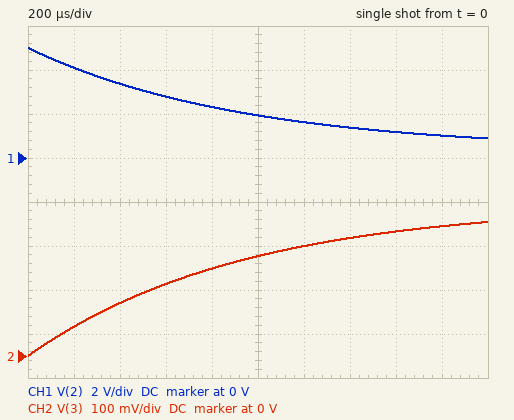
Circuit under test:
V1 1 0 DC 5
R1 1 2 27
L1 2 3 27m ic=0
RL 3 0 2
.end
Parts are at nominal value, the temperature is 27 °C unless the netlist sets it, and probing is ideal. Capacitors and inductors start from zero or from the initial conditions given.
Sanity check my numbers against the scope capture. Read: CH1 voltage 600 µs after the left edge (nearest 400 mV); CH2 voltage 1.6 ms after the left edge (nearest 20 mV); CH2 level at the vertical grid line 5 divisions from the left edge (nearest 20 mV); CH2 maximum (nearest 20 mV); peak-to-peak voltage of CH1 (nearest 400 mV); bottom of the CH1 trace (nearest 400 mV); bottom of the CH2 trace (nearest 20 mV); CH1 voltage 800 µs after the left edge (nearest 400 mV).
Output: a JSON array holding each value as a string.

["2.8 V", "280 mV", "220 mV", "300 mV", "4.0 V", "800 mV", "0 V", "2.4 V"]
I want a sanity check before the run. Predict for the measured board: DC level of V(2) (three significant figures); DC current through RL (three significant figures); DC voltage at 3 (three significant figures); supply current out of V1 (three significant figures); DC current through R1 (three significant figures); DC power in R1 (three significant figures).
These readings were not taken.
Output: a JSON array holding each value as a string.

["345 mV", "172 mA", "345 mV", "172 mA", "172 mA", "803 mW"]
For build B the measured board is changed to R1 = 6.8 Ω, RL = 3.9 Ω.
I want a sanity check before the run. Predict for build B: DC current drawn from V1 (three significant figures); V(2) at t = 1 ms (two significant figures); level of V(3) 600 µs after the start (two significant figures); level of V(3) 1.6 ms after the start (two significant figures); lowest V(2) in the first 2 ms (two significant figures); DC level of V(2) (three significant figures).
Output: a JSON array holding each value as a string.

["467 mA", "4.0 V", "390 mV", "860 mV", "3.3 V", "1.82 V"]
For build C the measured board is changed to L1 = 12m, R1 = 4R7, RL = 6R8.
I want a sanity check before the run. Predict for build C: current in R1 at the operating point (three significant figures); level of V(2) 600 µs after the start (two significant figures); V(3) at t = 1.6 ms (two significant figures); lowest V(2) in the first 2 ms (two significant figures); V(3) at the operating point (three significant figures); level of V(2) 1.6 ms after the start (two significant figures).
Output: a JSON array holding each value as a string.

["435 mA", "4.1 V", "2.3 V", "3.3 V", "2.96 V", "3.4 V"]
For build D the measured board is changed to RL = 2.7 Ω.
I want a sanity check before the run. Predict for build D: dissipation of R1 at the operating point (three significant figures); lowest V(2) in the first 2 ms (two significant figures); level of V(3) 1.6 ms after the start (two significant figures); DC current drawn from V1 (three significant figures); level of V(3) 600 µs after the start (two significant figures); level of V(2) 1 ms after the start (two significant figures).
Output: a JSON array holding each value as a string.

["765 mW", "960 mV", "380 mV", "168 mA", "220 mV", "2.0 V"]
